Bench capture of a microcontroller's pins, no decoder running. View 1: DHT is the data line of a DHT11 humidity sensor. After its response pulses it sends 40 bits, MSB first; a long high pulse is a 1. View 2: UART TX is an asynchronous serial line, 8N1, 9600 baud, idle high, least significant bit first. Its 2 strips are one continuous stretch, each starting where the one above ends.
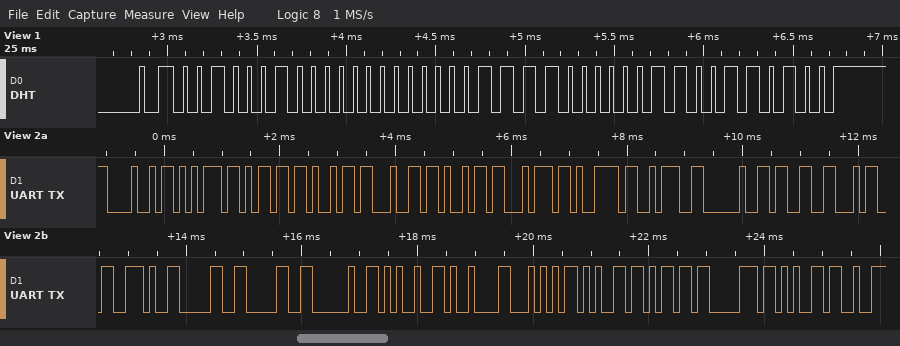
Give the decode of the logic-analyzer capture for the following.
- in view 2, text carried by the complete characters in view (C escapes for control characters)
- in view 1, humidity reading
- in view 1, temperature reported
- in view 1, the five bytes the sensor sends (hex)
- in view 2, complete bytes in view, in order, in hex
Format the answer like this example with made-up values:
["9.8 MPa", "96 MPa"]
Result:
["\"Humidity: 34.00 %\\tTempe\"", "34 %", "15.3 °C", "22 00 0F 03 34", "48 75 6D 69 64 69 74 79 3A 20 33 34 2E 30 30 20 25 09 54 65 6D 70 65"]
